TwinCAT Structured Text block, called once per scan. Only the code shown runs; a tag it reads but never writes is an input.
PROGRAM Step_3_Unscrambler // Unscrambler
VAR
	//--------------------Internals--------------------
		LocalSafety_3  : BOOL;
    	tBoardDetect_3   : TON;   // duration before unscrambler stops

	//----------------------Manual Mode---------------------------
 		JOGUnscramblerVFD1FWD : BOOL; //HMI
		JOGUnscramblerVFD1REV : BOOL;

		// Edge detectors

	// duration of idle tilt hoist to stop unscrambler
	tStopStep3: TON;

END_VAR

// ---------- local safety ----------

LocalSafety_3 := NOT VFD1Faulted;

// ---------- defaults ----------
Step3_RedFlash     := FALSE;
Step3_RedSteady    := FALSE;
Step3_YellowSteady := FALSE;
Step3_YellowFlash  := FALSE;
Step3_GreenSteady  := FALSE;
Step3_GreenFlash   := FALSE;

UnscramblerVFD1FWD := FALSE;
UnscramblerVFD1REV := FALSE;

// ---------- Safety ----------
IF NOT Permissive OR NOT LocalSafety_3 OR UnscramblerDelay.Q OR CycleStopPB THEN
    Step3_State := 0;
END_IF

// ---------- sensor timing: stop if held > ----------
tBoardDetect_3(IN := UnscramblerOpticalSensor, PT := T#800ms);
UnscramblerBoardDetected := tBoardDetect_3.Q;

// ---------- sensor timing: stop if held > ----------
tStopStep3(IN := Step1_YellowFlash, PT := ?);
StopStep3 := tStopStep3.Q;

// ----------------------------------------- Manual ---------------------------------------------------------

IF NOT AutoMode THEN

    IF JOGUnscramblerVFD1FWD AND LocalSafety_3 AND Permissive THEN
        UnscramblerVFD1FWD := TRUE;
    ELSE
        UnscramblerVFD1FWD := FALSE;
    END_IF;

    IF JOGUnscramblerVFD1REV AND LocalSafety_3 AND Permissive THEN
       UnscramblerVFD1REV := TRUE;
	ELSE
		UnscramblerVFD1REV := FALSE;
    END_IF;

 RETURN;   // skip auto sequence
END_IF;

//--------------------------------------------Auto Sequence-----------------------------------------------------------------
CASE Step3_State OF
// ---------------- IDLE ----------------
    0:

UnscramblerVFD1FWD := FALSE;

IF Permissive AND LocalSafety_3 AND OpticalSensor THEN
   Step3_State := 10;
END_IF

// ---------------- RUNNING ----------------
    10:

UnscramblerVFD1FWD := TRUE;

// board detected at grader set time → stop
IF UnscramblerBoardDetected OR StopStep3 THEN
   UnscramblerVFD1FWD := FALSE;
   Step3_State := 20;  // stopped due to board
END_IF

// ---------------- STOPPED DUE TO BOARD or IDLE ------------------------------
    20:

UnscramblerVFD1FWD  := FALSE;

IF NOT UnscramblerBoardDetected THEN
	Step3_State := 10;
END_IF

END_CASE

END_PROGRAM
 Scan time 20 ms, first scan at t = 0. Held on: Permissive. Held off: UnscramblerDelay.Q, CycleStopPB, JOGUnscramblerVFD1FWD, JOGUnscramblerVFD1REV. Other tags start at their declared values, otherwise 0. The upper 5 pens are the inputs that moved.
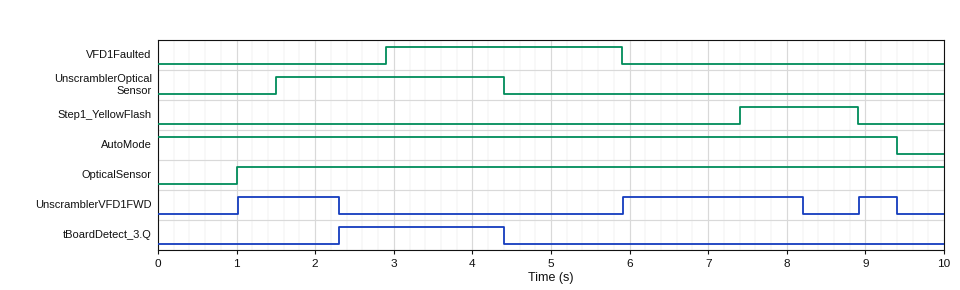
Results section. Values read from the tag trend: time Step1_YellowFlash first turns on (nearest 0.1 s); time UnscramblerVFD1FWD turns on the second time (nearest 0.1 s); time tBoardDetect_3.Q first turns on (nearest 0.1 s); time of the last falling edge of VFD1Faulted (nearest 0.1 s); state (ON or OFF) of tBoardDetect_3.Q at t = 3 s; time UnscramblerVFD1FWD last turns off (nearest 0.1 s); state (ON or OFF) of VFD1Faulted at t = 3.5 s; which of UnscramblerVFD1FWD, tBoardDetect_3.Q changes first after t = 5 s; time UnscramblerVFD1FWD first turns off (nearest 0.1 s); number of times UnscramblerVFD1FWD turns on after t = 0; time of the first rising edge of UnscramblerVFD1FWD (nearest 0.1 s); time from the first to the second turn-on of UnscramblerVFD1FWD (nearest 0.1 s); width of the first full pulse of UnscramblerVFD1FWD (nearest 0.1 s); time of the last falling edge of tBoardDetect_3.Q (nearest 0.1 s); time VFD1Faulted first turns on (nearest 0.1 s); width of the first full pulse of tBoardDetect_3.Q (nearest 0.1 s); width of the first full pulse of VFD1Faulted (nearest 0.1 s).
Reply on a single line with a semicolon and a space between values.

7.4 s; 5.9 s; 2.3 s; 5.9 s; ON; 9.4 s; ON; UnscramblerVFD1FWD; 2.3 s; 3; 1.0 s; 4.9 s; 1.3 s; 4.4 s; 2.9 s; 2.1 s; 3.0 s
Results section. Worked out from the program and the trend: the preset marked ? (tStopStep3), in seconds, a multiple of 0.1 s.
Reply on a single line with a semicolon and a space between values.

0.8 s
